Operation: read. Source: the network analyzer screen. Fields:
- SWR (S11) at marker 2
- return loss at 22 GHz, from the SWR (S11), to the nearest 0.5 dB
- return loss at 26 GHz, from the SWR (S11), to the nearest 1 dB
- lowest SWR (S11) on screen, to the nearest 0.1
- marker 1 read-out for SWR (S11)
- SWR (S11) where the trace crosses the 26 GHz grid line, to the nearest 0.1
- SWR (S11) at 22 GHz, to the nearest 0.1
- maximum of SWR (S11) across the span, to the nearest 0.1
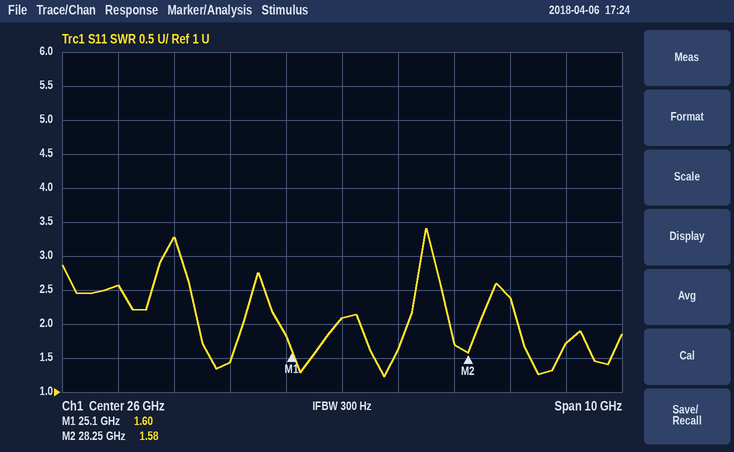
1.58
7.0 dB
9 dB
1.2
1.60
2.1
2.6
3.4
